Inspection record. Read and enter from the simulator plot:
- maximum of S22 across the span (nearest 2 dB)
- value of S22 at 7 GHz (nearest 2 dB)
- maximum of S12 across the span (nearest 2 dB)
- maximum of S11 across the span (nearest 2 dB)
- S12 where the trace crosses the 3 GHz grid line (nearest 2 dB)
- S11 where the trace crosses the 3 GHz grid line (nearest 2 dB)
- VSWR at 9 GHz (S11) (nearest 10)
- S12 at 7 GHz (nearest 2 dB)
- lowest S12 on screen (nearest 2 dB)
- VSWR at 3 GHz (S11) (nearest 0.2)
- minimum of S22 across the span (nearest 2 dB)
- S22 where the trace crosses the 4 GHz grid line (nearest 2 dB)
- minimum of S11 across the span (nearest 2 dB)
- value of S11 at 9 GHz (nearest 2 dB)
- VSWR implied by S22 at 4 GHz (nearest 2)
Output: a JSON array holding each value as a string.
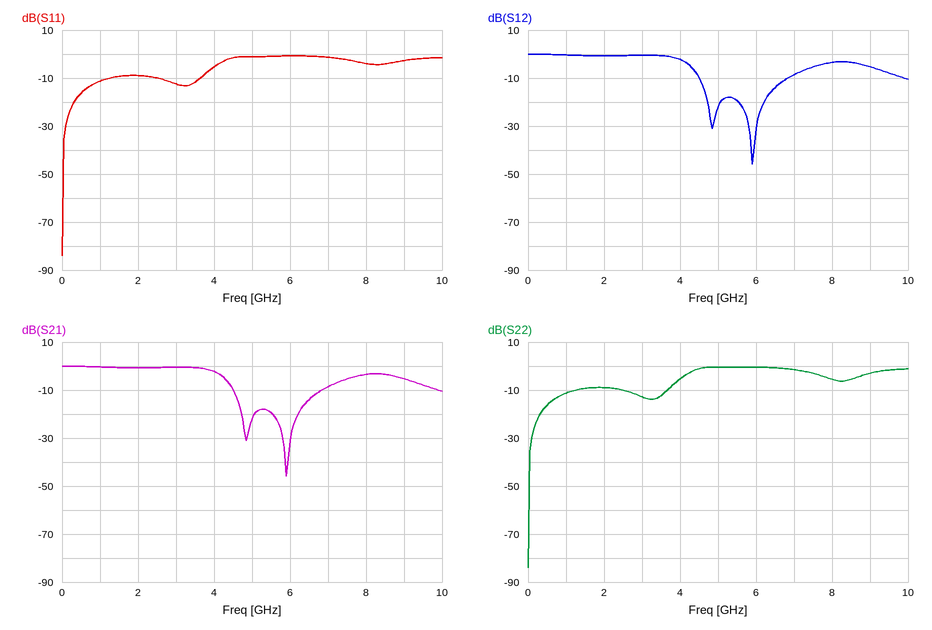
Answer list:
["0 dB", "-2 dB", "0 dB", "0 dB", "0 dB", "-12 dB", "10", "-8 dB", "-46 dB", "1.6", "-84 dB", "-6 dB", "-84 dB", "-2 dB", "4"]
